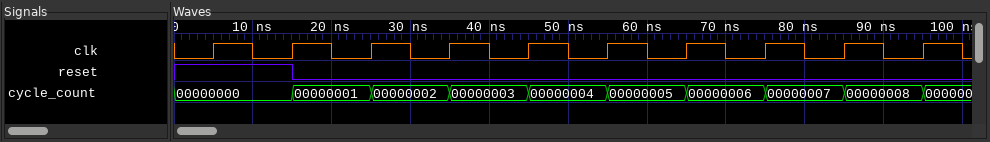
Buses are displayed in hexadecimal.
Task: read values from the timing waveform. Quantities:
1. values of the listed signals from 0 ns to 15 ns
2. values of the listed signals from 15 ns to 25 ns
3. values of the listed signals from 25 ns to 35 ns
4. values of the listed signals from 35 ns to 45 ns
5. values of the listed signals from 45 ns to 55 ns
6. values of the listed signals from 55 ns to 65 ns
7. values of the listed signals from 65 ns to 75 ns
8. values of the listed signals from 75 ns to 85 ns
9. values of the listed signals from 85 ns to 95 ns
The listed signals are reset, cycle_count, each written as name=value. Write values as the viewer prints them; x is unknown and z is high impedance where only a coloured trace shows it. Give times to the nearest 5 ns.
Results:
reset=1, cycle_count=00000000
reset=0, cycle_count=00000001
reset=0, cycle_count=00000002
reset=0, cycle_count=00000003
reset=0, cycle_count=00000004
reset=0, cycle_count=00000005
reset=0, cycle_count=00000006
reset=0, cycle_count=00000007
reset=0, cycle_count=00000008
